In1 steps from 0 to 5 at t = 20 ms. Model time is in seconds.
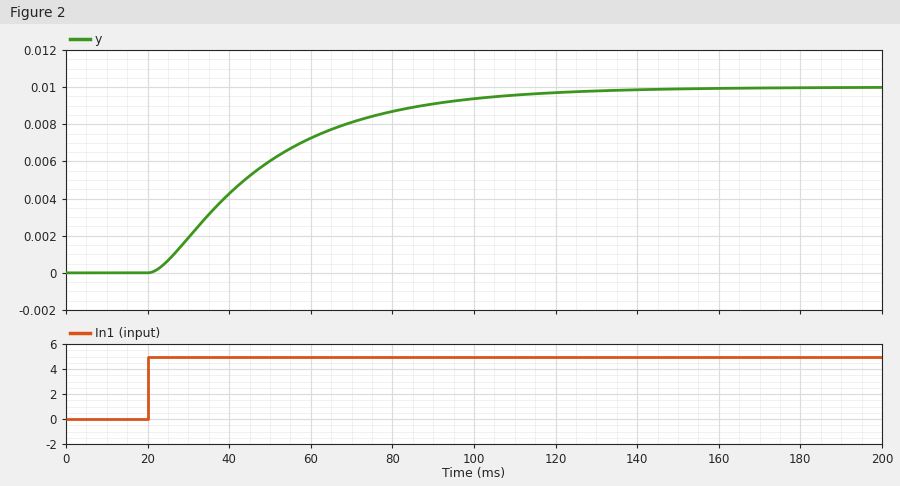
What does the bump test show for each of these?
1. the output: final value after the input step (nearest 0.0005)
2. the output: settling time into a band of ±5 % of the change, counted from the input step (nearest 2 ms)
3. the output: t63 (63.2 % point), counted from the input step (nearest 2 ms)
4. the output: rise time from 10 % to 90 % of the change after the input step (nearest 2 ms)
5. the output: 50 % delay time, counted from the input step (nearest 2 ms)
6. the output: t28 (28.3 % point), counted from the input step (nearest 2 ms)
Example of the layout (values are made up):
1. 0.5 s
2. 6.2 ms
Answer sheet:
1. 0.0100
2. 86 ms
3. 32 ms
4. 60 ms
5. 24 ms
6. 14 ms
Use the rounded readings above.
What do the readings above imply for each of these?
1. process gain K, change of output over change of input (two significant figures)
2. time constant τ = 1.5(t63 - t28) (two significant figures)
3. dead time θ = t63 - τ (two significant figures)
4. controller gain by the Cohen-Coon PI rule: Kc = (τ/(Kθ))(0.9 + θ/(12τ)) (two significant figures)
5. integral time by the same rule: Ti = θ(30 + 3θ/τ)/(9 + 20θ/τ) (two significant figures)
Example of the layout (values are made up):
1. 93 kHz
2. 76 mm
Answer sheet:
1. 0.0020
2. 27 ms
3. 5.0 ms
4. 2500
5. 12 ms
